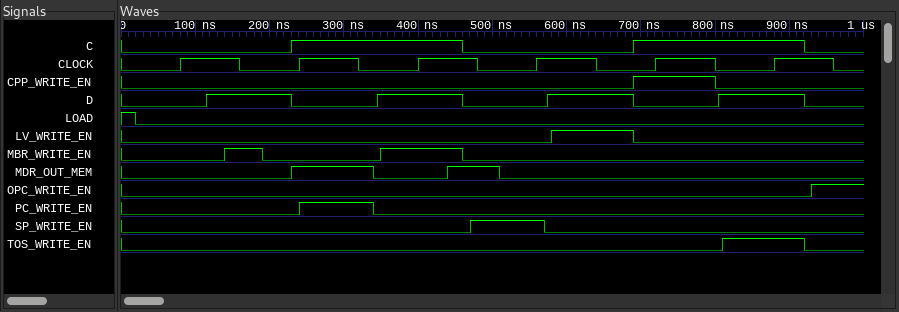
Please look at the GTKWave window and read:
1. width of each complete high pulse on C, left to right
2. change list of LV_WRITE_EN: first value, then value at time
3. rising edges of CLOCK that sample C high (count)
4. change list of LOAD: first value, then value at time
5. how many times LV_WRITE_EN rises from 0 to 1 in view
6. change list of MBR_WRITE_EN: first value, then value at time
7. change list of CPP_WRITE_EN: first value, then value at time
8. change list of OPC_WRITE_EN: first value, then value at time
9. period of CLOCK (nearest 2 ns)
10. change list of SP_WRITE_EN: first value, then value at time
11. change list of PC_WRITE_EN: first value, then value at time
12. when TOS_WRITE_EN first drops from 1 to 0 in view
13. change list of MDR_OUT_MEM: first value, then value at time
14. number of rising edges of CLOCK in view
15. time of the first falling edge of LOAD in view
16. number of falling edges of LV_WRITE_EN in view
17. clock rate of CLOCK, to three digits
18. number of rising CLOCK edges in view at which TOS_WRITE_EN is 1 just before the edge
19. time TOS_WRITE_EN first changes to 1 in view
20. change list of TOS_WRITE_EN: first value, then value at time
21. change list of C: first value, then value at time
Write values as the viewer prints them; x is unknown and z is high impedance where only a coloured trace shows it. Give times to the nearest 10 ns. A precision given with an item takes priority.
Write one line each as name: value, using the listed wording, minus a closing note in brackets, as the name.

width of each complete high pulse on C, left to right: 230 ns, 230 ns
change list of LV_WRITE_EN: first value, then value at time: 0, 1 at 580 ns, 0 at 690 ns
rising edges of CLOCK that sample C high: 4
change list of LOAD: first value, then value at time: 1, 0 at 20 ns
how many times LV_WRITE_EN rises from 0 to 1 in view: 1
change list of MBR_WRITE_EN: first value, then value at time: 0, 1 at 140 ns, 0 at 190 ns, 1 at 350 ns, 0 at 460 ns
change list of CPP_WRITE_EN: first value, then value at time: 0, 1 at 690 ns, 0 at 800 ns
change list of OPC_WRITE_EN: first value, then value at time: 0, 1 at 930 ns
period of CLOCK: 160 ns
change list of SP_WRITE_EN: first value, then value at time: 0, 1 at 470 ns, 0 at 570 ns
change list of PC_WRITE_EN: first value, then value at time: 0, 1 at 240 ns, 0 at 340 ns
when TOS_WRITE_EN first drops from 1 to 0 in view: 920 ns
change list of MDR_OUT_MEM: first value, then value at time: 0, 1 at 230 ns, 0 at 340 ns, 1 at 440 ns, 0 at 510 ns
number of rising edges of CLOCK in view: 6
time of the first falling edge of LOAD in view: 20 ns
number of falling edges of LV_WRITE_EN in view: 1
clock rate of CLOCK, to three digits: 6.25 MHz
number of rising CLOCK edges in view at which TOS_WRITE_EN is 1 just before the edge: 1
time TOS_WRITE_EN first changes to 1 in view: 810 ns
change list of TOS_WRITE_EN: first value, then value at time: 0, 1 at 810 ns, 0 at 920 ns
change list of C: first value, then value at time: 0, 1 at 230 ns, 0 at 460 ns, 1 at 690 ns, 0 at 920 ns
